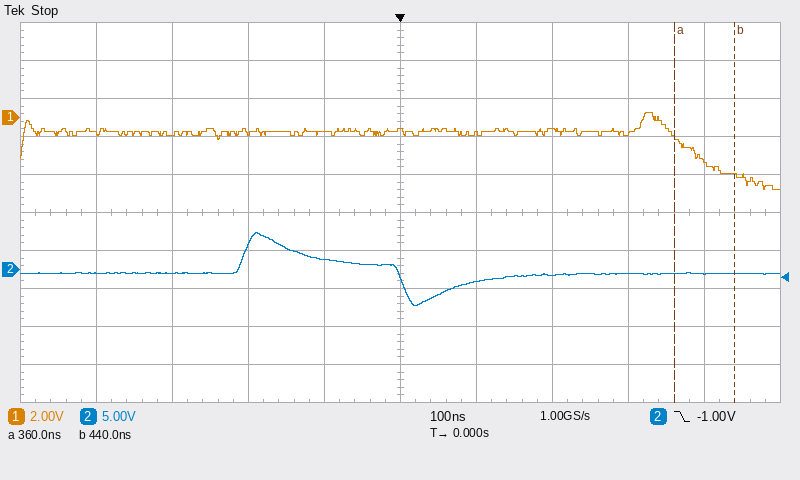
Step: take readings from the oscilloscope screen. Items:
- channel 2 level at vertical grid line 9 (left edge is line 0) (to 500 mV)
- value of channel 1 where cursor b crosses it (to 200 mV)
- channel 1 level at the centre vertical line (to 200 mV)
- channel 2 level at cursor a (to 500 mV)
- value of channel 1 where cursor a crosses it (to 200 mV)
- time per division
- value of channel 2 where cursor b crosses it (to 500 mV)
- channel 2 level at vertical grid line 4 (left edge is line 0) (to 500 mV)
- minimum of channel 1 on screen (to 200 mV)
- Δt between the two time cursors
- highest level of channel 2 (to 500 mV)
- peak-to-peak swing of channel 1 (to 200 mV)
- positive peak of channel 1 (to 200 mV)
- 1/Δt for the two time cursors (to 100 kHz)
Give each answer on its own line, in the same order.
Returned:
-500 mV
-3.0 V
-800 mV
-500 mV
-1.0 V
100 ns
-500 mV
1.5 V
-3.8 V
80 ns
5.0 V
4.0 V
200 mV
12.5 MHz
